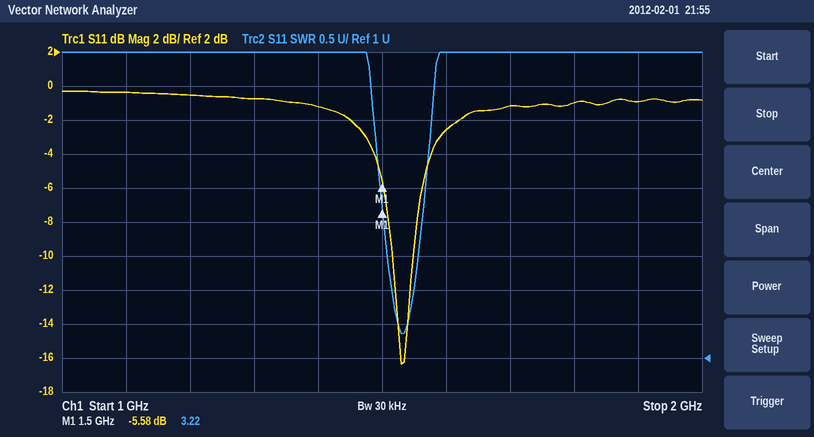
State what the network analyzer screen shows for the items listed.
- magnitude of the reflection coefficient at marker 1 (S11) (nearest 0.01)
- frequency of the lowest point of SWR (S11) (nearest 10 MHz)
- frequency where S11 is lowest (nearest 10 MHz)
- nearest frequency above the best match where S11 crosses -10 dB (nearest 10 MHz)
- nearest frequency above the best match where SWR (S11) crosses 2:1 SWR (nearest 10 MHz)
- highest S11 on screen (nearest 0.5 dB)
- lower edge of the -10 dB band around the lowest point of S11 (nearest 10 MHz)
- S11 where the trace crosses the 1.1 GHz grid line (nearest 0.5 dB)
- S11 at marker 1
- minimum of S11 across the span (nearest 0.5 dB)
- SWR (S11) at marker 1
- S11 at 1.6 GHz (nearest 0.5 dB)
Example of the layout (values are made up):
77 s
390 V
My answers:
0.53
1.53 GHz
1.53 GHz
1.55 GHz
1.55 GHz
-0.5 dB
1.52 GHz
-0.5 dB
-5.58 dB
-16.5 dB
3.22
-2.5 dB
